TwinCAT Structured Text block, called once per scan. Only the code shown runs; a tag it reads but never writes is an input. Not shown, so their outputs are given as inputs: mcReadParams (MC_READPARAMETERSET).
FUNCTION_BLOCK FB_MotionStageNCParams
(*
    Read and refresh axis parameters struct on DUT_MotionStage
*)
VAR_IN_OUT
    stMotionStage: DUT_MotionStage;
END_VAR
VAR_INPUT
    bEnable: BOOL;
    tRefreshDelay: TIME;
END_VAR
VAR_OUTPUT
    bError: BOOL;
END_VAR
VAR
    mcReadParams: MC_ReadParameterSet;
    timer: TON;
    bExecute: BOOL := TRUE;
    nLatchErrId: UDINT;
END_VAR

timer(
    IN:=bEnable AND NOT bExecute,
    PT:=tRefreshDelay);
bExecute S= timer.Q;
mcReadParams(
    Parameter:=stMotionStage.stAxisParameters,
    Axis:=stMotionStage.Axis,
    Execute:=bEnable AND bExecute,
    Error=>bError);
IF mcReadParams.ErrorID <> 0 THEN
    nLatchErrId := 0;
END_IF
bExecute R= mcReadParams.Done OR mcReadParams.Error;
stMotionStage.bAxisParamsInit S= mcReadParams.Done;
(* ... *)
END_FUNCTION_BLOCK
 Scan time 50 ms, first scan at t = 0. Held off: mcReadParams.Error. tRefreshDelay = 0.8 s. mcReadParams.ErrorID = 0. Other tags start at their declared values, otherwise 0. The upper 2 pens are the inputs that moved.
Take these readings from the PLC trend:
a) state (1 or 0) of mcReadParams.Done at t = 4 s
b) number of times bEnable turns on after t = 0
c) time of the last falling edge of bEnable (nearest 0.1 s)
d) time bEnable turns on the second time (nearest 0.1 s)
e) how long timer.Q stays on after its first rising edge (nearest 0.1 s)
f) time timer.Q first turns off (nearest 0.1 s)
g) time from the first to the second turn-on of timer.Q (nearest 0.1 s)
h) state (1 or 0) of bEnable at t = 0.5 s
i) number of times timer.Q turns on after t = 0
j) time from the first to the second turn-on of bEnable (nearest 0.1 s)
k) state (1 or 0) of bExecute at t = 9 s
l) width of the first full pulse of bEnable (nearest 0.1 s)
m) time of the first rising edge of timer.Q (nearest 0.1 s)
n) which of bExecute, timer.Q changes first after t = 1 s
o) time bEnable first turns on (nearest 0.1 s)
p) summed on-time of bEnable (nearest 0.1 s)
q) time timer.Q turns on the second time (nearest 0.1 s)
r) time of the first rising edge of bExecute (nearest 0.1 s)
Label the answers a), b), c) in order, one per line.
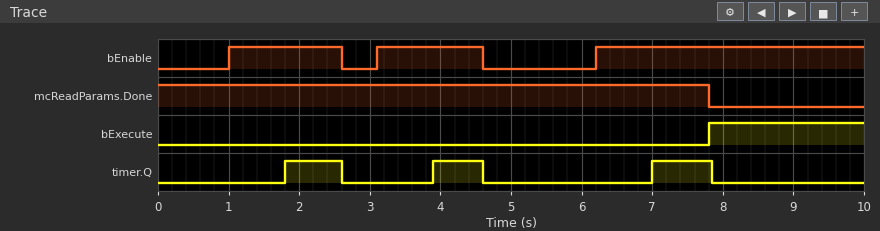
a) 1
b) 3
c) 4.6 s
d) 3.1 s
e) 0.8 s
f) 2.6 s
g) 2.1 s
h) 0
i) 3
j) 2.1 s
k) 1
l) 1.6 s
m) 1.8 s
n) timer.Q
o) 1.0 s
p) 6.9 s
q) 3.9 s
r) 7.8 s
